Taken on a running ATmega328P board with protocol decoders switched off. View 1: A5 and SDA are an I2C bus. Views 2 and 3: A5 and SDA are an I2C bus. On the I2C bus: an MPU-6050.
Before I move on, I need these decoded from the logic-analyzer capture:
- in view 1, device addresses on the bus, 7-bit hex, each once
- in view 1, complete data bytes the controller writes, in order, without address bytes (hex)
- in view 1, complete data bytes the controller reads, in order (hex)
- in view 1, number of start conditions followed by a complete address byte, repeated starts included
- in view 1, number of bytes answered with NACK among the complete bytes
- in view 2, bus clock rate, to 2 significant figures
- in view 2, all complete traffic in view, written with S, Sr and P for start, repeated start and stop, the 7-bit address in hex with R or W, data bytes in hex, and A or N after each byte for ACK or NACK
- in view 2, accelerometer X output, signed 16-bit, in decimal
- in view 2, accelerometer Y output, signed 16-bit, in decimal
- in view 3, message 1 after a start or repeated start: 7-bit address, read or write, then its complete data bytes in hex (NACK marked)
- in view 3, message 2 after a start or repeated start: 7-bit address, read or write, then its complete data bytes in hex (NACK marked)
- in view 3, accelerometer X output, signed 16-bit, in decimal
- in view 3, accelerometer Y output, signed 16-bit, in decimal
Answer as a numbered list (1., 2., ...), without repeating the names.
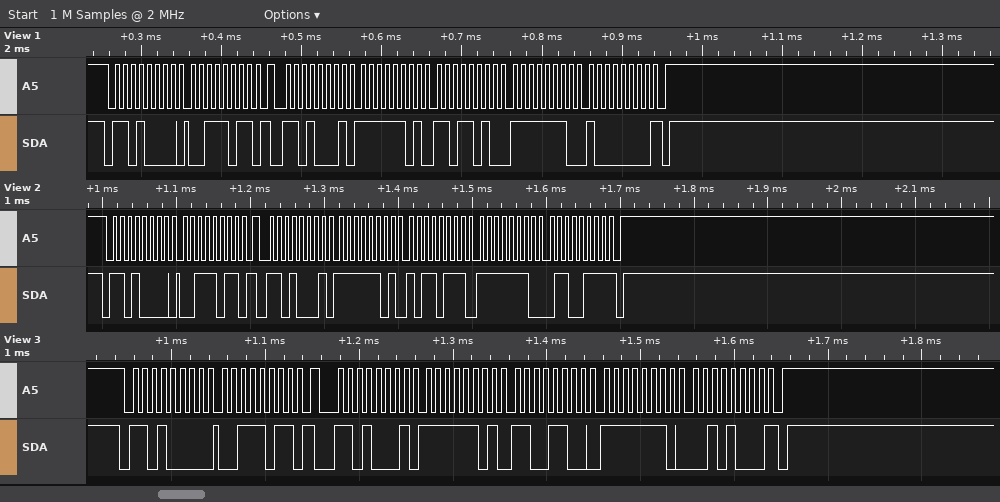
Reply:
1. 0x68
2. 3B
3. FD DA FE 80
4. 2
5. 1
6. 100 kHz
7. S 68W A 3B A Sr 68R A FD A B7 A FE A 67 N P
8. -585
9. -409
10. 0x68 write: 3B
11. 0x68 read: FD CC FE 28 NACK
12. -564
13. -472
